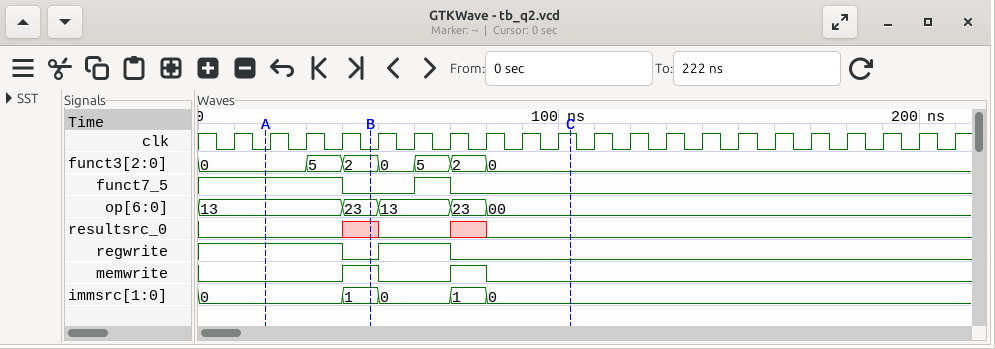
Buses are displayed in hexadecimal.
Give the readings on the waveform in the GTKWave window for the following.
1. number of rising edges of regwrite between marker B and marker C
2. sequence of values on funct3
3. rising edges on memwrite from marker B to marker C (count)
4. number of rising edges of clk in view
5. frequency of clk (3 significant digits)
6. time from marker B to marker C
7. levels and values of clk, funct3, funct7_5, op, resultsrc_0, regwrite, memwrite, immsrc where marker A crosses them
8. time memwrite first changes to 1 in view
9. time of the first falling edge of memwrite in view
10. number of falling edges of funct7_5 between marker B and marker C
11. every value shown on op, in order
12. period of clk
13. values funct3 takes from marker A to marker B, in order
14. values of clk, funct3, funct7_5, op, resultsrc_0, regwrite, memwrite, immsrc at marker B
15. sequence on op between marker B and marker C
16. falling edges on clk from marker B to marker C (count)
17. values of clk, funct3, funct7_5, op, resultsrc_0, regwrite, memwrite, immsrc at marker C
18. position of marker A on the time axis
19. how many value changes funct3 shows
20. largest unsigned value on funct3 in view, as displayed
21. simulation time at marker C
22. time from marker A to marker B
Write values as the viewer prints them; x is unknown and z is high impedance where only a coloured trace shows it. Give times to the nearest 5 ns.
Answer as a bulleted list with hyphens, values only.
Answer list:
- 1
- 0, 5, 2, 0, 5, 2, 0
- 1
- 21
- 100 MHz
- 55 ns
- clk=0, funct3=0, funct7_5=1, op=13, resultsrc_0=0, regwrite=1, memwrite=0, immsrc=0
- 40 ns
- 50 ns
- 1
- 13, 23, 13, 23, 00
- 10 ns
- 0, 5, 2
- clk=0, funct3=2, funct7_5=0, op=23, resultsrc_0=x, regwrite=0, memwrite=1, immsrc=1
- 23, 13, 23, 00
- 5
- clk=1, funct3=0, funct7_5=0, op=00, resultsrc_0=0, regwrite=0, memwrite=0, immsrc=0
- 20 ns
- 6
- 5
- 105 ns
- 30 ns
